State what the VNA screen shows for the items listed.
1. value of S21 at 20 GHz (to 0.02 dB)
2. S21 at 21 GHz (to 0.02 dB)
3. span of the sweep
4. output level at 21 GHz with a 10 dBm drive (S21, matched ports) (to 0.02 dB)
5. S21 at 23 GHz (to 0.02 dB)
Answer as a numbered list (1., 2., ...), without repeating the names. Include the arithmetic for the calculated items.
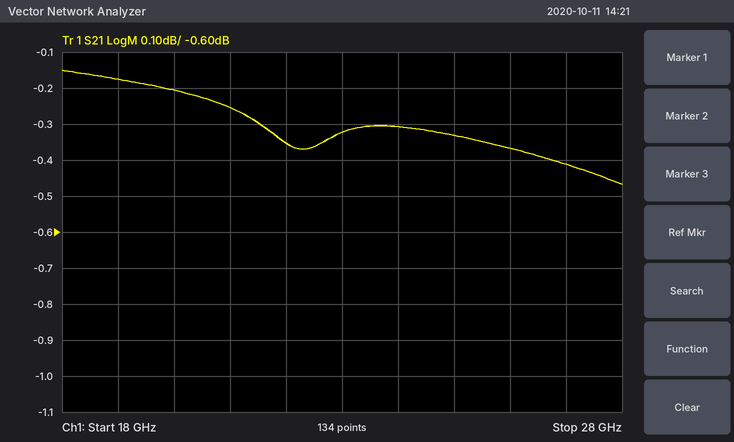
1. -0.20 dB
2. -0.26 dB
3. 10 GHz
4. 10 dBm + (-0.26 dB) = 9.74 dBm
5. -0.32 dB
